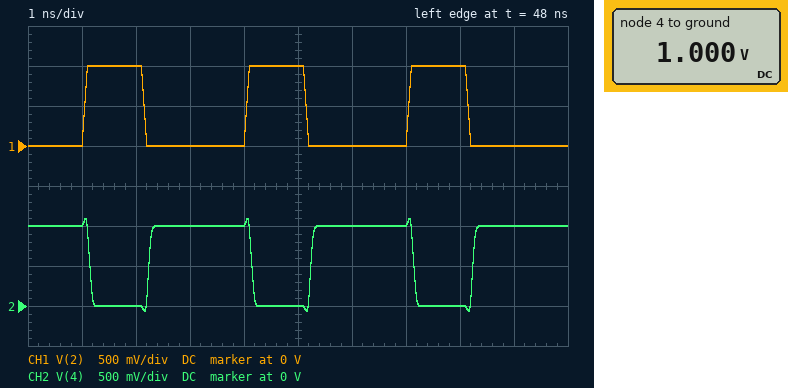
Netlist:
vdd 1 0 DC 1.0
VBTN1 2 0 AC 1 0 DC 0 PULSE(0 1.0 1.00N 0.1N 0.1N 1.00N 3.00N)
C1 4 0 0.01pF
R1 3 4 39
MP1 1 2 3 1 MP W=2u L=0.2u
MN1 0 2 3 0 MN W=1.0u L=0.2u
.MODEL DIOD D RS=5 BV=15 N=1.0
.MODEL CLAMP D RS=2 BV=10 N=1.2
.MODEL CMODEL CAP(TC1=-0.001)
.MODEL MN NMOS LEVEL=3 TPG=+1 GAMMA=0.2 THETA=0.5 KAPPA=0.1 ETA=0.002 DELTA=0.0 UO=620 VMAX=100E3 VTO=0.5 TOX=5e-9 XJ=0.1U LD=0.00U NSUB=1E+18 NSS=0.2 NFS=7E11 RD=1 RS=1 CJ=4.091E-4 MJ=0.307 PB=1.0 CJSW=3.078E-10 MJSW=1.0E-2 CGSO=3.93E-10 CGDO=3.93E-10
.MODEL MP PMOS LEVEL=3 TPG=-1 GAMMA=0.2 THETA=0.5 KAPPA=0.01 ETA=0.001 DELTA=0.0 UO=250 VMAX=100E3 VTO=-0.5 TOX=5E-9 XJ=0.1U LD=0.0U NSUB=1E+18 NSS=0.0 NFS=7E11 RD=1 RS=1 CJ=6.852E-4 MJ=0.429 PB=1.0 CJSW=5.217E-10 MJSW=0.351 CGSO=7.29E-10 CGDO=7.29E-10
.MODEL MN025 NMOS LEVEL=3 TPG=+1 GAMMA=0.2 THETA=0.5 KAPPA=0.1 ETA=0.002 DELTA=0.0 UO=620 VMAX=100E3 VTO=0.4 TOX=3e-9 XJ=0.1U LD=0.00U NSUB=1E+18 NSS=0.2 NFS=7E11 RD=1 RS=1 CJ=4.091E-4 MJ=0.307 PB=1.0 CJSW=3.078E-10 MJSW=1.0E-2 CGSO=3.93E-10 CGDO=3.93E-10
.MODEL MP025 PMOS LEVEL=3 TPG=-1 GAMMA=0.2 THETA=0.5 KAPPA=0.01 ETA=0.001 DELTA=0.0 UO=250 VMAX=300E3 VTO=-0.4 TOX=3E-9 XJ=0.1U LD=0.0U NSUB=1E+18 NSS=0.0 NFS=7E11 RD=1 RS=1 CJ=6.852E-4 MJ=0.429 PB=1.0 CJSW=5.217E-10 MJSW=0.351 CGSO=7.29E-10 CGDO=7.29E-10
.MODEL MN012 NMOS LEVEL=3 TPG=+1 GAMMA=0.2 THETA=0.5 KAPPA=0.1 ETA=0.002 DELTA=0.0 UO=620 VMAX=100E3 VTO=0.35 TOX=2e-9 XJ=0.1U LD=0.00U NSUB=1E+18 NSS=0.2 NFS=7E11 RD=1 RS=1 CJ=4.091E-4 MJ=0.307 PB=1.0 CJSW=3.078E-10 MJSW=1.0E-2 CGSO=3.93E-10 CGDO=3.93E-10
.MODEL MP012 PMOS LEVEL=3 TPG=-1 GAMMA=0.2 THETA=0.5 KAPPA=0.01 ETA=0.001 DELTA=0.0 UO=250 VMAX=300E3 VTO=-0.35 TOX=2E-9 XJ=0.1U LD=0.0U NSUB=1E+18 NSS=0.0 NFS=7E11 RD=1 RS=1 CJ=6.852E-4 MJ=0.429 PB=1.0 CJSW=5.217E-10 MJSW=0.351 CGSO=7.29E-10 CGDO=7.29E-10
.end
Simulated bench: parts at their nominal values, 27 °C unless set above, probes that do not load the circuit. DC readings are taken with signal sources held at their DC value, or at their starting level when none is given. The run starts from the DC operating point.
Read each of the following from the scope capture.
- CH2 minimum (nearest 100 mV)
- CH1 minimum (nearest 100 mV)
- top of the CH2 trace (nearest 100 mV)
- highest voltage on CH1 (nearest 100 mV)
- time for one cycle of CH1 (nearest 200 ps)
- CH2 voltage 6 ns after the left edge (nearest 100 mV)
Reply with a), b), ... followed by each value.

a) -100 mV
b) 0 V
c) 1.1 V
d) 1.0 V
e) 3.0 ns
f) 1.0 V
